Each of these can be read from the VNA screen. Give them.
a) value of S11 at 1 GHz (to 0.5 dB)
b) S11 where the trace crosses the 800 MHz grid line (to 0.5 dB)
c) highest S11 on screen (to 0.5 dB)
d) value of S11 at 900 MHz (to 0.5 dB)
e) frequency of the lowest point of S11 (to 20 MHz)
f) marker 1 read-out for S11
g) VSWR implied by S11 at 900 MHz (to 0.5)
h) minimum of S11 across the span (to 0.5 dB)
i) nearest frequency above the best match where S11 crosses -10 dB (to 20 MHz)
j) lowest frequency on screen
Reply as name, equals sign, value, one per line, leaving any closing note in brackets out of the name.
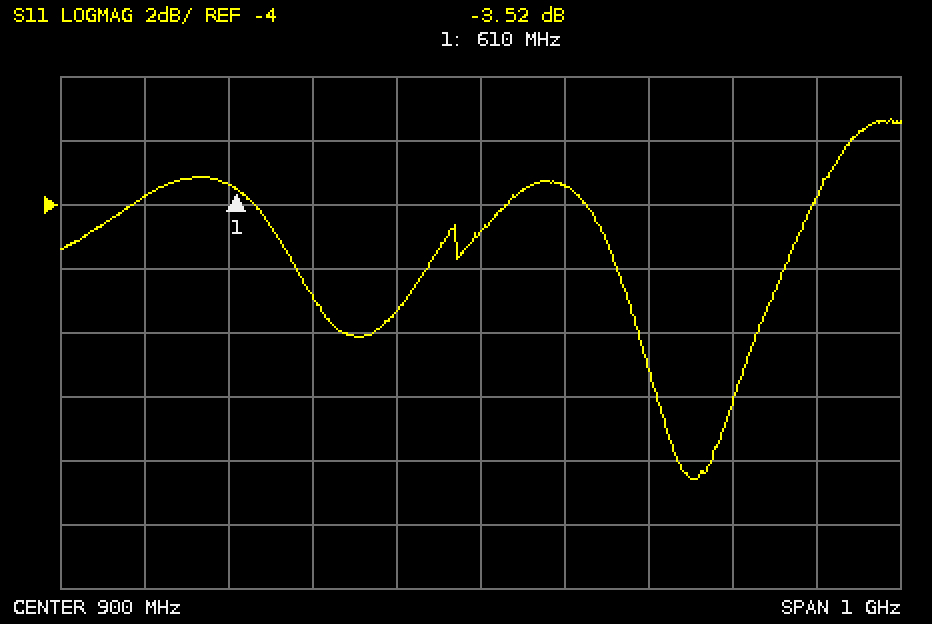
value of S11 at 1 GHz = -3.5 dB
S11 where the trace crosses the 800 MHz grid line = -7.5 dB
highest S11 on screen = -1.5 dB
value of S11 at 900 MHz = -5.0 dB
frequency of the lowest point of S11 = 1.16 GHz
marker 1 read-out for S11 = -3.52 dB
VSWR implied by S11 at 900 MHz = 3.5
minimum of S11 across the span = -12.5 dB
nearest frequency above the best match where S11 crosses -10 dB = 1.20 GHz
lowest frequency on screen = 400 MHz
